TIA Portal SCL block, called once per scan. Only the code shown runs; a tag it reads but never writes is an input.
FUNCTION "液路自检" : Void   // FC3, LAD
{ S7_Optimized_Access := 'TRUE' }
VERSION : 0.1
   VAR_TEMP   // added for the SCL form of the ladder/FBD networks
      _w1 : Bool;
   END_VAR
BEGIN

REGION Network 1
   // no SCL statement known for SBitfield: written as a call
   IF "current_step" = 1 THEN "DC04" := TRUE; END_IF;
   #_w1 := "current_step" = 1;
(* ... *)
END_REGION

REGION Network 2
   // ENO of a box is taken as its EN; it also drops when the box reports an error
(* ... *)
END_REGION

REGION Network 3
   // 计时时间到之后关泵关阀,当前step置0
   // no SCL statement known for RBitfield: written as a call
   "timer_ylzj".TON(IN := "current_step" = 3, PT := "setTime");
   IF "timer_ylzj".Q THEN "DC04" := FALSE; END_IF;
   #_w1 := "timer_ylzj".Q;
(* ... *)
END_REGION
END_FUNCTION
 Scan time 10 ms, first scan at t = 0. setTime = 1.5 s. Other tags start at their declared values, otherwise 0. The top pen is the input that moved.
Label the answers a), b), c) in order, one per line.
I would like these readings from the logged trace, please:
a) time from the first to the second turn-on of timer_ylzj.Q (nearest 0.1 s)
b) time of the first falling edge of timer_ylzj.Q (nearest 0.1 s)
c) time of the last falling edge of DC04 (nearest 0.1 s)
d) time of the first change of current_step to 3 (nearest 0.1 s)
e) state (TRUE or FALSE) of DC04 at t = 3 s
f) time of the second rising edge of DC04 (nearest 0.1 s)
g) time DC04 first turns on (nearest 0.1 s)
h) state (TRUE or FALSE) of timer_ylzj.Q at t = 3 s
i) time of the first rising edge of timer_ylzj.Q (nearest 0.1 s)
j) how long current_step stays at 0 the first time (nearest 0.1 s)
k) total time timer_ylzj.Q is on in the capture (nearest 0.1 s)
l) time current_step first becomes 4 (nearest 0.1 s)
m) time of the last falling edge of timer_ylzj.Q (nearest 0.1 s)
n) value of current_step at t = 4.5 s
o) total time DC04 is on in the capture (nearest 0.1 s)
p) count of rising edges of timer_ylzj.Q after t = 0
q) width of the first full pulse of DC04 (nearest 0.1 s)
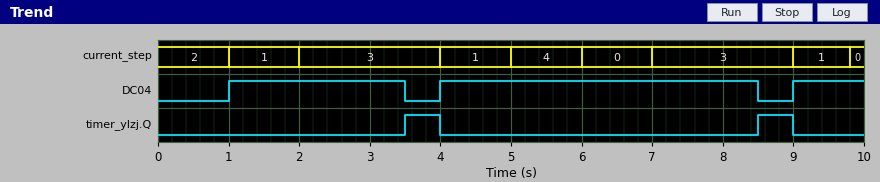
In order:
a) 5.0 s
b) 4.0 s
c) 8.5 s
d) 2.0 s
e) TRUE
f) 4.0 s
g) 1.0 s
h) FALSE
i) 3.5 s
j) 1.0 s
k) 1.0 s
l) 5.0 s
m) 9.0 s
n) 1
o) 8.0 s
p) 2
q) 2.5 s
